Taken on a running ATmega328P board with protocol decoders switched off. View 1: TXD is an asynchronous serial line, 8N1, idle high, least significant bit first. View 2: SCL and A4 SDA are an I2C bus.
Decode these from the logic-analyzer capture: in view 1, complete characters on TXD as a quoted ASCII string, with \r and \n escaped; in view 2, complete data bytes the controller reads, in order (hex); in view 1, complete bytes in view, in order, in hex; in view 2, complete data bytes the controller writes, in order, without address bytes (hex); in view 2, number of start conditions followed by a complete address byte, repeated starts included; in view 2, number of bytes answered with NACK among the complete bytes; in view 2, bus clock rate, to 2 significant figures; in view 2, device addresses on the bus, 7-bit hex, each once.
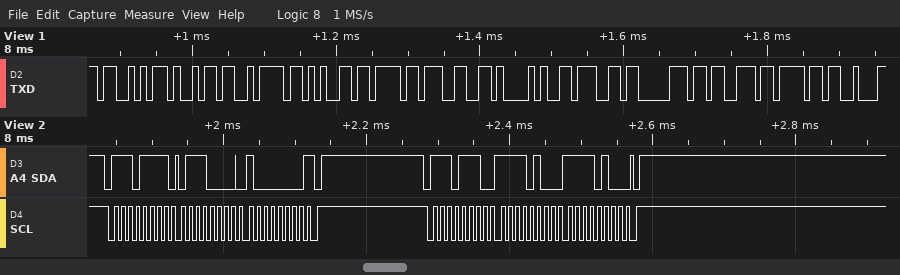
"Sizeof(gpso"
70 80
53 69 7A 65 6F 66 28 67 70 73 6F
F4 F4
2
1
100 kHz
0x77
